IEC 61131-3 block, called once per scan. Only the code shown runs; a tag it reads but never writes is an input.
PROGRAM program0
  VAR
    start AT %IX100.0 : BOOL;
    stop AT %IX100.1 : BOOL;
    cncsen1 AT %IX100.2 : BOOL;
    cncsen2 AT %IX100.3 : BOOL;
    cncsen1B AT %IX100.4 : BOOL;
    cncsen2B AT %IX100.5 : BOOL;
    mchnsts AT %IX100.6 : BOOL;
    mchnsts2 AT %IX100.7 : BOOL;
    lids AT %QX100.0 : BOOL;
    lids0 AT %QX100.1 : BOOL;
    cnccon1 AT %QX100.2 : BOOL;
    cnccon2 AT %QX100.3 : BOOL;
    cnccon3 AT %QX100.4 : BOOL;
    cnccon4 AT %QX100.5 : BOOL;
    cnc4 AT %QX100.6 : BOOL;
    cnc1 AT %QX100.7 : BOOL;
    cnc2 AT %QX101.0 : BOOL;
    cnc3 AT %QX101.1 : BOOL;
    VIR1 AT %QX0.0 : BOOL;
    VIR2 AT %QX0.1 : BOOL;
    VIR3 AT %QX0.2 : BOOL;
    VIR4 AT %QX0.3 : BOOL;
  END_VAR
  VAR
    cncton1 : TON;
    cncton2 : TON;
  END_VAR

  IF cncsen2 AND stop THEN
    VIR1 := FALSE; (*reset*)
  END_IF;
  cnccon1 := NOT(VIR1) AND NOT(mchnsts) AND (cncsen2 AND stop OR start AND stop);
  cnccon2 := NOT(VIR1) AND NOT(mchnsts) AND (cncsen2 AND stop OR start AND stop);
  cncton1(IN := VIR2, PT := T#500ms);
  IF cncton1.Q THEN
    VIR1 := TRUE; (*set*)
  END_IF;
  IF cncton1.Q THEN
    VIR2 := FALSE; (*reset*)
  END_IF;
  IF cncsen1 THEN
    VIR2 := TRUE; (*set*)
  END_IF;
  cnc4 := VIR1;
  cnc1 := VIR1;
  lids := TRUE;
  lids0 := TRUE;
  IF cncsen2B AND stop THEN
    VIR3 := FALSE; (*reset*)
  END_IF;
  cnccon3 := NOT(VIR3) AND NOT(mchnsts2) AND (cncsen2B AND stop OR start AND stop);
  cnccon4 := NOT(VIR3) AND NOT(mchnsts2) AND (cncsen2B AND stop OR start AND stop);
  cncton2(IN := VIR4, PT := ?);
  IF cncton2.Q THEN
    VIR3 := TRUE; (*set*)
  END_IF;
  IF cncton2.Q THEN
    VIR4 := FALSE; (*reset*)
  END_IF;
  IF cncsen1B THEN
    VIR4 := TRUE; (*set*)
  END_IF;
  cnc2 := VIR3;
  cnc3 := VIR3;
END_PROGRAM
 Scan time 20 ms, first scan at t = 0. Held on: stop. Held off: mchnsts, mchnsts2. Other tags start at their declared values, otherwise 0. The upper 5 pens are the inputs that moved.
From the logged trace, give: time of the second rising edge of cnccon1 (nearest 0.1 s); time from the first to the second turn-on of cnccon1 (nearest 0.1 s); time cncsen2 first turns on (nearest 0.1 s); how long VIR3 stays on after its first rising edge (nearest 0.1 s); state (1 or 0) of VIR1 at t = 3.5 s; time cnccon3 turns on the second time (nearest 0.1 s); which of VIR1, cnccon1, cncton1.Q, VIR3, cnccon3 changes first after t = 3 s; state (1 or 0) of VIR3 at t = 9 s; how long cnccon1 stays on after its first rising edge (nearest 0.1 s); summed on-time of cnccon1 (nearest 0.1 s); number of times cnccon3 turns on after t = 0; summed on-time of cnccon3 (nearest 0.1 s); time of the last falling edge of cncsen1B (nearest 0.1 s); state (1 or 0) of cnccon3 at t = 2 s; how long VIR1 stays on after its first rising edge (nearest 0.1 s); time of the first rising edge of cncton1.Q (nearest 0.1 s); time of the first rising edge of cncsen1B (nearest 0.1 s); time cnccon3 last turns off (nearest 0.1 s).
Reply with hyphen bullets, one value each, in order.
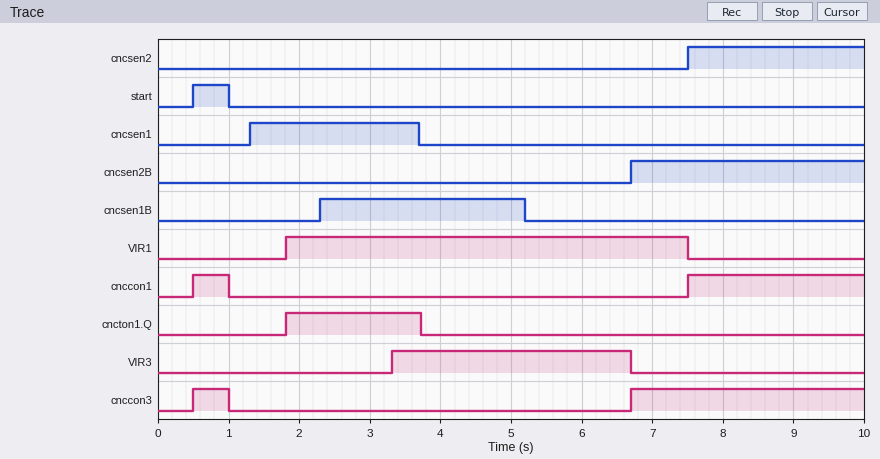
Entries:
- 7.5 s
- 7.0 s
- 7.5 s
- 3.4 s
- 1
- 6.7 s
- VIR3
- 0
- 0.5 s
- 3.0 s
- 2
- 3.8 s
- 5.2 s
- 0
- 5.7 s
- 1.8 s
- 2.3 s
- 1.0 s
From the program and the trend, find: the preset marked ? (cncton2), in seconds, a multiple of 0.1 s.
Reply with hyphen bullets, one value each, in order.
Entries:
- 1.0 s
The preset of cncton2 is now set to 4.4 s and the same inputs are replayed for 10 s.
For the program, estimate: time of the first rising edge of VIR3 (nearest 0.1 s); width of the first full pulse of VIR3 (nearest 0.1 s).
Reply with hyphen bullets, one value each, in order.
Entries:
- 6.7 s
- 0.0 s
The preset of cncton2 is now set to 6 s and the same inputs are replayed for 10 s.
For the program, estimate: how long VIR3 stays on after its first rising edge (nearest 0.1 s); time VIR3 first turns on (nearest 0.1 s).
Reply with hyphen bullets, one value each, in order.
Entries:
- 0.0 s
- 8.3 s
